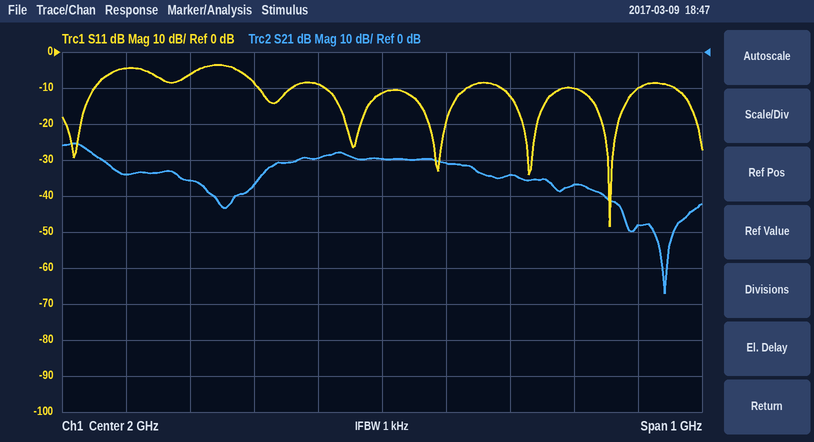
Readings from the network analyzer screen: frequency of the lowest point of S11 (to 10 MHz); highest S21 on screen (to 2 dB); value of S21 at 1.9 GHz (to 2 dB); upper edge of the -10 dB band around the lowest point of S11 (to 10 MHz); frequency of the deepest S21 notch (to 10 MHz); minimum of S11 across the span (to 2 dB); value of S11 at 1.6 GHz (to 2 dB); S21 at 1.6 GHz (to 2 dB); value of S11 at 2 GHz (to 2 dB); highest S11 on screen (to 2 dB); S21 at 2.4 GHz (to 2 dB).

2.36 GHz
-26 dB
-30 dB
2.40 GHz
2.44 GHz
-48 dB
-4 dB
-34 dB
-12 dB
-4 dB
-48 dB
